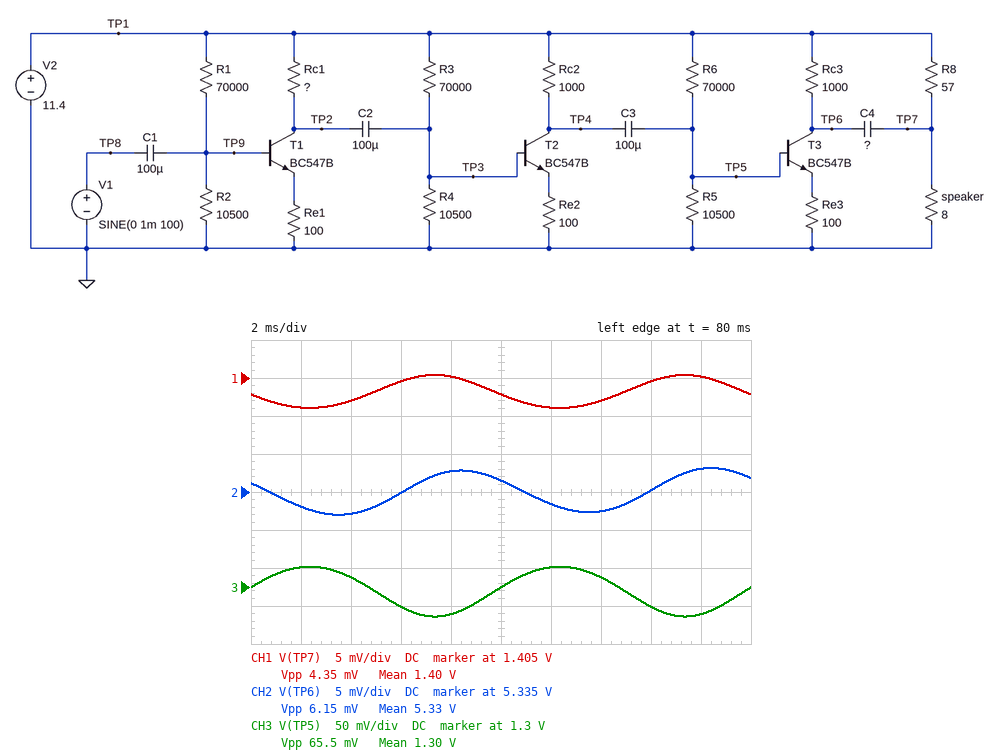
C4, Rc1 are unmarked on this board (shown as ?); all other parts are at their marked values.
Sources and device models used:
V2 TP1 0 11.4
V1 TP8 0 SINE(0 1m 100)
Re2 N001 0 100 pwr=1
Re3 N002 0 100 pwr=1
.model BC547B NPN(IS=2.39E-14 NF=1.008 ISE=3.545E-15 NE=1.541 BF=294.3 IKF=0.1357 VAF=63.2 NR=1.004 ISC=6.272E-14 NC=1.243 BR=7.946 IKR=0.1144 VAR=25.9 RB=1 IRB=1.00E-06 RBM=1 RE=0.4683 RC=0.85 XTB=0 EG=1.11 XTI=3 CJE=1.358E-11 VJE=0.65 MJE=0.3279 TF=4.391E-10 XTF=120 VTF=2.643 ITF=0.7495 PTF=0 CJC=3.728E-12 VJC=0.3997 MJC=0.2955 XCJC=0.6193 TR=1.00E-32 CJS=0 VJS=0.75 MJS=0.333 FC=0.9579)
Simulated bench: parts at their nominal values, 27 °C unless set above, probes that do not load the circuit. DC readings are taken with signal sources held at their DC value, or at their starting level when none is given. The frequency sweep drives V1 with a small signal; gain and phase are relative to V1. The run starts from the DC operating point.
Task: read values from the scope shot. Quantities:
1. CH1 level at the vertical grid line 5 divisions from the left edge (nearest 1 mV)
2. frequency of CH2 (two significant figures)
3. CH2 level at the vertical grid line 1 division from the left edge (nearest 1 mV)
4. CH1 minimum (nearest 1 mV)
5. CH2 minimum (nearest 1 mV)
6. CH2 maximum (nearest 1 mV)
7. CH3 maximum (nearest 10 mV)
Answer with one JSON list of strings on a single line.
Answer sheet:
["1.403 V", "100 Hz", "5.333 V", "1.401 V", "5.332 V", "5.338 V", "1.33 V"]
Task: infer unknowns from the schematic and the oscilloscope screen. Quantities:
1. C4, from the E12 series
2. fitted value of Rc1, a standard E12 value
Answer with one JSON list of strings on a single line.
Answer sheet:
["270 µF", "2.7 kΩ"]
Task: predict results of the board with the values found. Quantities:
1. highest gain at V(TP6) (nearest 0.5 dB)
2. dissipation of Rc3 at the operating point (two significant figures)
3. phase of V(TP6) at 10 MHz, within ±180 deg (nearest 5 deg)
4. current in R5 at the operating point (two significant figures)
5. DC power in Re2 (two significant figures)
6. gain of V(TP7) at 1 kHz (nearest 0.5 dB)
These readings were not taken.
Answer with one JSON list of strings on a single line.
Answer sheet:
["26.0 dB", "37 mW", "60 deg", "120 µA", "3.7 mW", "6.5 dB"]
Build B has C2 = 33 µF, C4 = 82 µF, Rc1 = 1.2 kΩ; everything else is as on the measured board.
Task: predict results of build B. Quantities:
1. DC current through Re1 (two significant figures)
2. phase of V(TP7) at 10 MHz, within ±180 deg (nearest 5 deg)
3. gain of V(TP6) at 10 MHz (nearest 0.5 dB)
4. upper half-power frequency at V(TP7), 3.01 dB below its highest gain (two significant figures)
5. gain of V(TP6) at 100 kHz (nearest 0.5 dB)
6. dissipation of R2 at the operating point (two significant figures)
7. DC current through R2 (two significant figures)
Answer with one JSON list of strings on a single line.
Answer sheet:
["6.1 mA", "95 deg", "7.0 dB", "4.7 MHz", "14.5 dB", "160 µW", "120 µA"]
